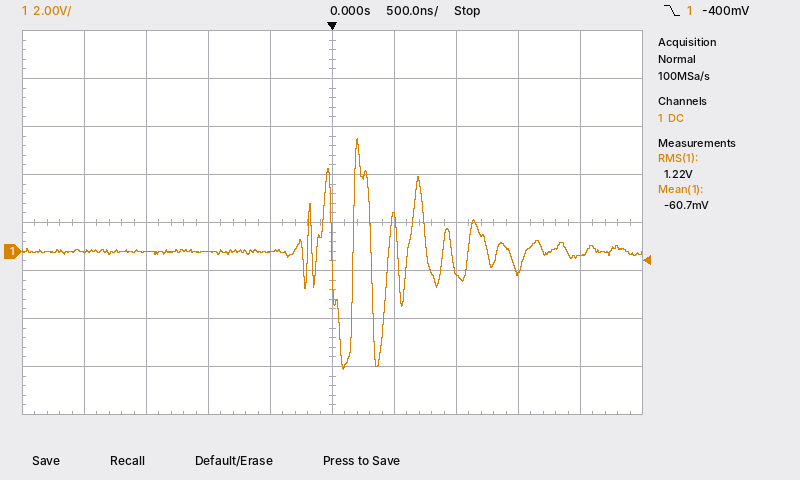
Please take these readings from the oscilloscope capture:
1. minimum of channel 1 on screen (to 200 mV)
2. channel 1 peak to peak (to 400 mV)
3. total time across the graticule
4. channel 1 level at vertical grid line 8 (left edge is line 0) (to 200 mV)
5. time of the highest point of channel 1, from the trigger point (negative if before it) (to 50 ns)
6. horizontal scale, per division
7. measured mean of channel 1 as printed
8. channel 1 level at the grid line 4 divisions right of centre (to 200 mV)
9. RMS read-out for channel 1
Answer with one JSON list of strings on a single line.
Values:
["-5.0 V", "9.6 V", "5 µs", "-800 mV", "+200 ns", "500 ns", "-60.7 mV", "-200 mV", "1.22 V"]
